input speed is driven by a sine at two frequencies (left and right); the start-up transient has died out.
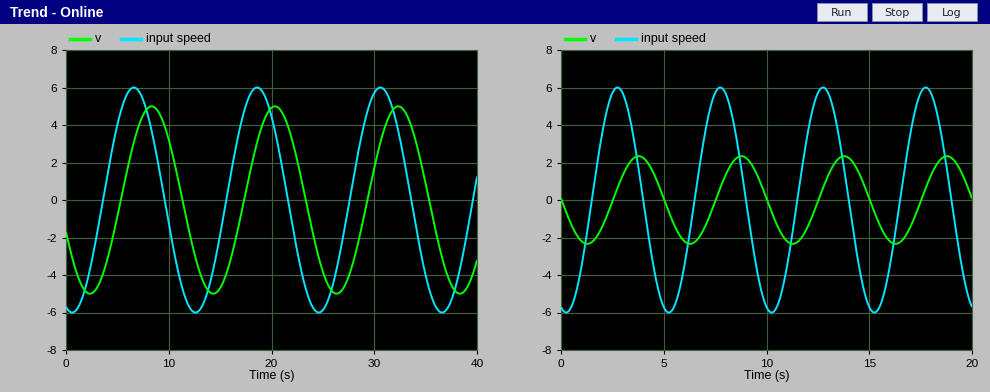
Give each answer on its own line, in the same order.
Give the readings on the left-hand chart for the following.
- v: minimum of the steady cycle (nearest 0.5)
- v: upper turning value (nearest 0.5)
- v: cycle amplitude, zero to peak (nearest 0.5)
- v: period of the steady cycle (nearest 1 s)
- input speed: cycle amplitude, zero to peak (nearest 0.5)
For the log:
-5.0
5.0
5.0
12 s
6.0
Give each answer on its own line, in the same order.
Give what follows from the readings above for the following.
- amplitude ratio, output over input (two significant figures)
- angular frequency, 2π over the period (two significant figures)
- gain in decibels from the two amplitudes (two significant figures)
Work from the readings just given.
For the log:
0.83
0.52 rad/s
-1.6 dB
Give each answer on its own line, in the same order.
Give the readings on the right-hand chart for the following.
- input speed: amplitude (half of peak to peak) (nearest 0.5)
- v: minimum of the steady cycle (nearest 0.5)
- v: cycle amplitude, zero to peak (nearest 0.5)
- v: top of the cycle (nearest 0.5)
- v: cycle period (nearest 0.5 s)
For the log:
6.0
-2.5
2.5
2.5
5.0 s
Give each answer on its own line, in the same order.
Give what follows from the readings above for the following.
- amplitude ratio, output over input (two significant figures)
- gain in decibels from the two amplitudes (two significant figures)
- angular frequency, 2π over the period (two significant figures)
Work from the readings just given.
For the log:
0.42
-7.6 dB
1.3 rad/s
